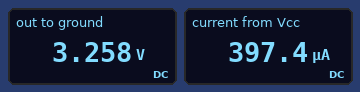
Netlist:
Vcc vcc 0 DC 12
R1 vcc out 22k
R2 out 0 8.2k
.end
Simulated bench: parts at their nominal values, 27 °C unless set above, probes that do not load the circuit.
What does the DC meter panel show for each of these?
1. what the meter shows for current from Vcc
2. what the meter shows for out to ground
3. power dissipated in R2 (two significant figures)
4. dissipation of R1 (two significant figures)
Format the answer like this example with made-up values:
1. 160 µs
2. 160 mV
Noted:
1. 397.4 µA
2. 3.258 V
3. 1.3 mW
4. 3.5 mW
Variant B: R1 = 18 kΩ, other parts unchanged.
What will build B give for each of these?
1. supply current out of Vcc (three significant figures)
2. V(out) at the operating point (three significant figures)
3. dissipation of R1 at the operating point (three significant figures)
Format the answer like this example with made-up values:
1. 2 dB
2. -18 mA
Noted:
1. 458 µA
2. 3.76 V
3. 3.78 mW
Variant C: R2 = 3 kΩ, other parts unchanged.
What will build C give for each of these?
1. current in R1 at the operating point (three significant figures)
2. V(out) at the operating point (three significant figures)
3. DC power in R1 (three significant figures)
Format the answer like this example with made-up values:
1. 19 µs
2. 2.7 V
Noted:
1. 480 µA
2. 1.44 V
3. 5.07 mW
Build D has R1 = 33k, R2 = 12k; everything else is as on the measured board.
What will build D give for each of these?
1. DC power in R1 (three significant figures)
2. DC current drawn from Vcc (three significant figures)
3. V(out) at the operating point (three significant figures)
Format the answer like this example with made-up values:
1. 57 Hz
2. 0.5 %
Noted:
1. 2.35 mW
2. 267 µA
3. 3.20 V
